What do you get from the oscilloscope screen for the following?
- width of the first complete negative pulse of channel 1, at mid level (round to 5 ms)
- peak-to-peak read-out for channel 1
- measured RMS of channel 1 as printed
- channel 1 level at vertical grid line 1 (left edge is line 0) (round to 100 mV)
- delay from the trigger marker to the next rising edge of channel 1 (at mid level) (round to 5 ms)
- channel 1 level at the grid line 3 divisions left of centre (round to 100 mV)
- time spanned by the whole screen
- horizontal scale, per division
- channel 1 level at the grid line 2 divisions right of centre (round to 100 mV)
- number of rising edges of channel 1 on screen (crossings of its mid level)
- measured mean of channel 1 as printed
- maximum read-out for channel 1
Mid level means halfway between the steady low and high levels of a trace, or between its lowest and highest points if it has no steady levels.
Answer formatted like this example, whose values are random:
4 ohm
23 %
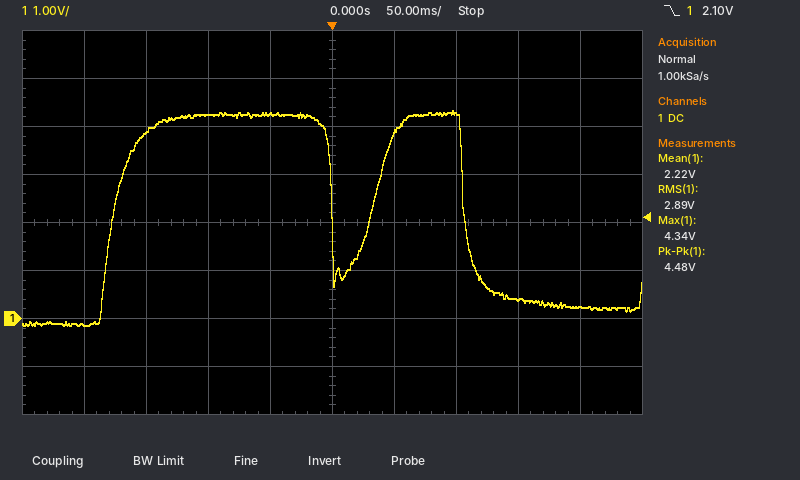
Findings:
30 ms
4.48 V
2.89 V
-100 mV
30 ms
3.9 V
500 ms
50 ms
4.3 V
2
2.22 V
4.34 V
